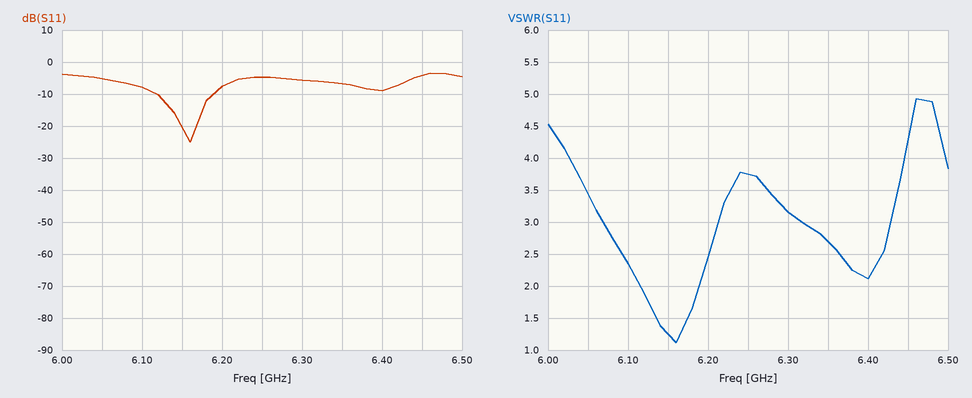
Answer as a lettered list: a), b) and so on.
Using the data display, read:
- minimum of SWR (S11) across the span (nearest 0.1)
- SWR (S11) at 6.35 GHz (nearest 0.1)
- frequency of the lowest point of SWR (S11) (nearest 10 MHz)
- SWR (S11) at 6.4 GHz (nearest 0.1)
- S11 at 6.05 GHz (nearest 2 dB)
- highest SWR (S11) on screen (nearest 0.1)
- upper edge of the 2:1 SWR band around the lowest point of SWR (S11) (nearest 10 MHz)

a) 1.1
b) 2.7
c) 6.16 GHz
d) 2.1
e) -6 dB
f) 4.9
g) 6.19 GHz
